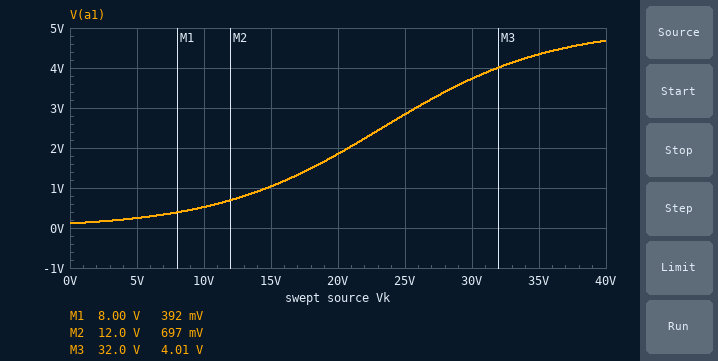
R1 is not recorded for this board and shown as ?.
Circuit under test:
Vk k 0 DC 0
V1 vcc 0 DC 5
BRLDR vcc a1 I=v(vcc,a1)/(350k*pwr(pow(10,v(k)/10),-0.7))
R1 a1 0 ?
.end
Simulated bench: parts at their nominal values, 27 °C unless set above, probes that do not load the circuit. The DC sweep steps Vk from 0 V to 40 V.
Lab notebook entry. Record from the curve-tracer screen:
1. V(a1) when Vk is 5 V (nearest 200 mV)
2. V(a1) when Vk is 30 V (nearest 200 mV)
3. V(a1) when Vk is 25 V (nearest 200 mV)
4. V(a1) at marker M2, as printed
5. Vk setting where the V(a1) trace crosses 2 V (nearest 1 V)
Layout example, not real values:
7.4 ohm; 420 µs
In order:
200 mV; 3.8 V; 2.8 V; 697 mV; 21 V
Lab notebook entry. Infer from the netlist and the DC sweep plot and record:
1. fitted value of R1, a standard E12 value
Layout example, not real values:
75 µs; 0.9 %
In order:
8.2 kΩ
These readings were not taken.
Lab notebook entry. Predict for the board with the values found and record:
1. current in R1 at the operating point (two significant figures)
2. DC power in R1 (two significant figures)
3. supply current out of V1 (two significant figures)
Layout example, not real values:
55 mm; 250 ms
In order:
14 µA; 1.6 µW; 14 µA
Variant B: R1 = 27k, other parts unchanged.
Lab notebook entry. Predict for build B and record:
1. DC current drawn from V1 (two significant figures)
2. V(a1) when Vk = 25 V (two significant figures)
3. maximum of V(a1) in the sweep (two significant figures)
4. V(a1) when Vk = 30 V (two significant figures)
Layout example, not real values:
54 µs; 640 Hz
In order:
13 µA; 4.1 V; 4.9 V; 4.5 V
